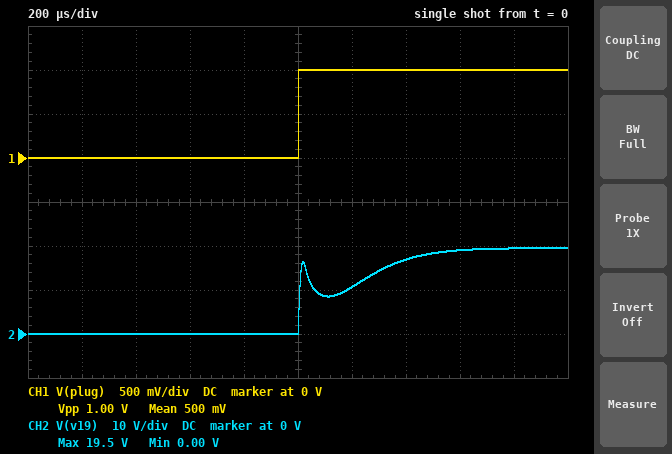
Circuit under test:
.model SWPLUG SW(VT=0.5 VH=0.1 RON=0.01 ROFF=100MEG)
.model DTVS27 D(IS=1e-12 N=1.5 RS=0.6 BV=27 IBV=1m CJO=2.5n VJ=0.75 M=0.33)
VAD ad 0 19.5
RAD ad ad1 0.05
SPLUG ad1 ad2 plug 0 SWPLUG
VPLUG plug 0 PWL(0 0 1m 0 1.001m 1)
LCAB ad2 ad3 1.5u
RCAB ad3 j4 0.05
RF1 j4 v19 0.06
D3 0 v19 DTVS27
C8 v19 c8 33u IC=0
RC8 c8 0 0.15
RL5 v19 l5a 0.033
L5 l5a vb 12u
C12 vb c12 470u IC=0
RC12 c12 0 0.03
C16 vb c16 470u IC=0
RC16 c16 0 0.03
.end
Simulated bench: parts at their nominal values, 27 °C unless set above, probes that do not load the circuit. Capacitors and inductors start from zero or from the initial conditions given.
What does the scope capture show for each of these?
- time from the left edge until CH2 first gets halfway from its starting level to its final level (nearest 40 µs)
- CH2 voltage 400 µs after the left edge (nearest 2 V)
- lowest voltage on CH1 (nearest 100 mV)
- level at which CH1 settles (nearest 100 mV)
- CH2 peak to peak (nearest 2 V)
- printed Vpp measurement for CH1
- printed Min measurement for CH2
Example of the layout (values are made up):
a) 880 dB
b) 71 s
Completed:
a) 1.00 ms
b) 0 V
c) 0 V
d) 1.0 V
e) 20 V
f) 1.00 V
g) 0.00 V
